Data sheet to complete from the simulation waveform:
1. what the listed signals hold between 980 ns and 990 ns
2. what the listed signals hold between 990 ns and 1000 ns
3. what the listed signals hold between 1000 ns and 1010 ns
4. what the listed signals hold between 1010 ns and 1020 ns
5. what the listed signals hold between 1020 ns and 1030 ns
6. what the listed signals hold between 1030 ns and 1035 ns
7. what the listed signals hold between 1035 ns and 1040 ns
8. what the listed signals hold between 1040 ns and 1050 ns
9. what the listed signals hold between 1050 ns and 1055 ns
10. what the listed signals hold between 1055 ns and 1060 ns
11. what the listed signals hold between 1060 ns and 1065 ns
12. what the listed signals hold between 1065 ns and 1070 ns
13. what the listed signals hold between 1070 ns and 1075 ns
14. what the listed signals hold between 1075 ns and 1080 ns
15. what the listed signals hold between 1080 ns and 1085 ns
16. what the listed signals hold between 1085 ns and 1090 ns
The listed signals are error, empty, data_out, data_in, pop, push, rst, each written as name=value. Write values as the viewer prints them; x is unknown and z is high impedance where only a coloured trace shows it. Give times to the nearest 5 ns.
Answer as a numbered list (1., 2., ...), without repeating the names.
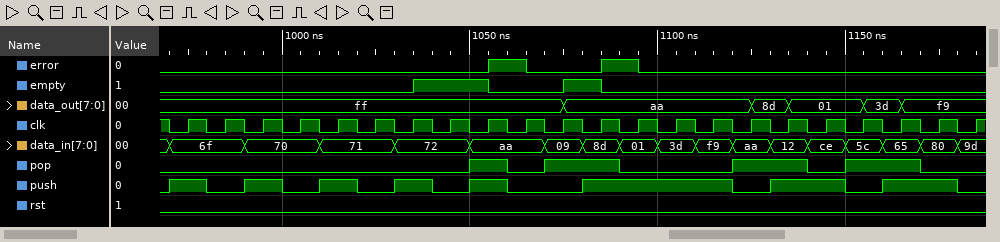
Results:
1. error=0, empty=0, data_out=ff, data_in=6f, pop=0, push=0, rst=0
2. error=0, empty=0, data_out=ff, data_in=70, pop=0, push=1, rst=0
3. error=0, empty=0, data_out=ff, data_in=70, pop=0, push=0, rst=0
4. error=0, empty=0, data_out=ff, data_in=71, pop=0, push=1, rst=0
5. error=0, empty=0, data_out=ff, data_in=71, pop=0, push=0, rst=0
6. error=0, empty=0, data_out=ff, data_in=72, pop=0, push=1, rst=0
7. error=0, empty=1, data_out=ff, data_in=72, pop=0, push=1, rst=0
8. error=0, empty=1, data_out=ff, data_in=72, pop=0, push=0, rst=0
9. error=0, empty=1, data_out=ff, data_in=aa, pop=1, push=1, rst=0
10. error=1, empty=0, data_out=ff, data_in=aa, pop=1, push=1, rst=0
11. error=1, empty=0, data_out=ff, data_in=aa, pop=0, push=0, rst=0
12. error=0, empty=0, data_out=ff, data_in=aa, pop=0, push=0, rst=0
13. error=0, empty=0, data_out=ff, data_in=09, pop=1, push=0, rst=0
14. error=0, empty=1, data_out=aa, data_in=09, pop=1, push=0, rst=0
15. error=0, empty=1, data_out=aa, data_in=8d, pop=1, push=1, rst=0
16. error=1, empty=0, data_out=aa, data_in=8d, pop=1, push=1, rst=0
